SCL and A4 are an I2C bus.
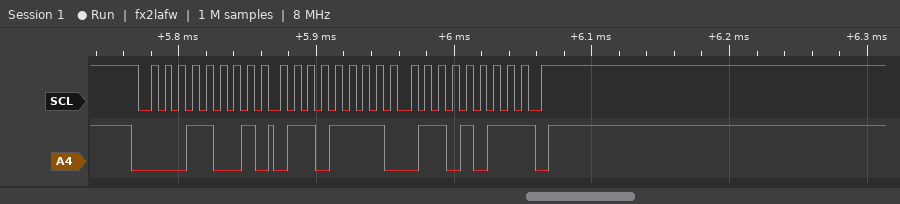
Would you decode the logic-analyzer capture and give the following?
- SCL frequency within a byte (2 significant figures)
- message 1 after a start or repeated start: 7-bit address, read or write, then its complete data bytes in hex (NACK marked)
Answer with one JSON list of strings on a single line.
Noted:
["100 kHz", "0x0C read: 6F 6B NACK"]
